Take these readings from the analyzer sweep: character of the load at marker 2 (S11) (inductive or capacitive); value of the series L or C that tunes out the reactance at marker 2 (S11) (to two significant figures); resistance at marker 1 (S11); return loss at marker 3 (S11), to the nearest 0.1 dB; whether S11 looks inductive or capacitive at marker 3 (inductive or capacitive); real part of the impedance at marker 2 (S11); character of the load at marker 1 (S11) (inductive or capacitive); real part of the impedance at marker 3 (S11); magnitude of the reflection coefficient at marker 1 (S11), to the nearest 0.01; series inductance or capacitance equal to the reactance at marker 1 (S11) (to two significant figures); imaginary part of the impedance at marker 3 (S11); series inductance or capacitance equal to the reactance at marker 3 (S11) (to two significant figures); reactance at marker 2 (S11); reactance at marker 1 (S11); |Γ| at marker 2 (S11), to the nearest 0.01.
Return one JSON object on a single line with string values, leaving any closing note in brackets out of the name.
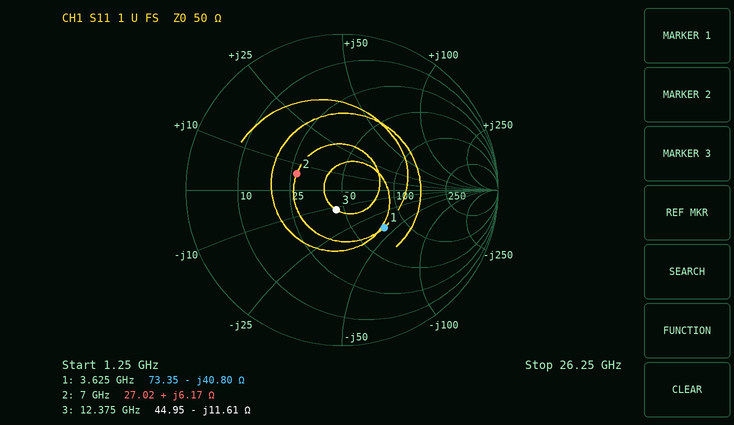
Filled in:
{"character of the load at marker 2 (S11)": "inductive", "value of the series L or C that tunes out the reactance at marker 2 (S11)": "3.7 pF", "resistance at marker 1": "73.35 Ω", "return loss at marker 3 (S11), to the nearest 0.1 dB": "17.6 dB", "whether S11 looks inductive or capacitive at marker 3": "capacitive", "real part of the impedance at marker 2": "27.02 Ω", "character of the load at marker 1 (S11)": "capacitive", "real part of the impedance at marker 3": "44.95 Ω", "magnitude of the reflection coefficient at marker 1 (S11), to the nearest 0.01": "0.36", "series inductance or capacitance equal to the reactance at marker 1 (S11)": "1.1 pF", "imaginary part of the impedance at marker 3": "-11.61 Ω", "series inductance or capacitance equal to the reactance at marker 3 (S11)": "1.1 pF", "reactance at marker 2": "+6.17 Ω", "reactance at marker 1": "-40.80 Ω", "|Γ| at marker 2 (S11), to the nearest 0.01": "0.31"}
